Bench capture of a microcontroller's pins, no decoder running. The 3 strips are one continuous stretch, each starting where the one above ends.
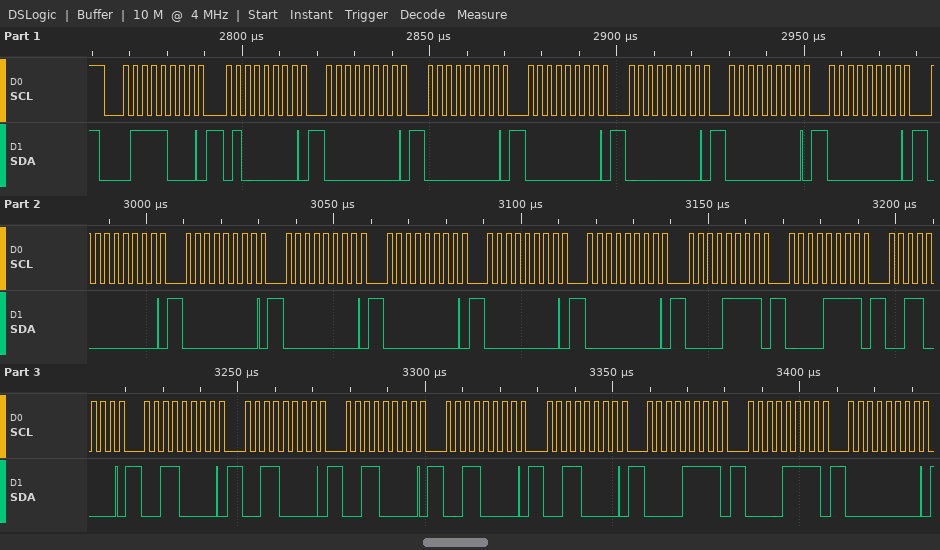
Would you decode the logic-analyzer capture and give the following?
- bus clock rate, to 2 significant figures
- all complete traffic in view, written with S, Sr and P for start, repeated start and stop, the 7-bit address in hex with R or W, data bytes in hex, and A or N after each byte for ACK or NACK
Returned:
400 kHz
S 3CW A 40 A 00 A 00 A 00 A 00 A 00 A 00 A 00 A 00 A 00 A 00 A 00 A 00 A 0F A 0F A 30 A 30 A 30 A 30 A 30 A 30 A 0F A 0F A 00 A
